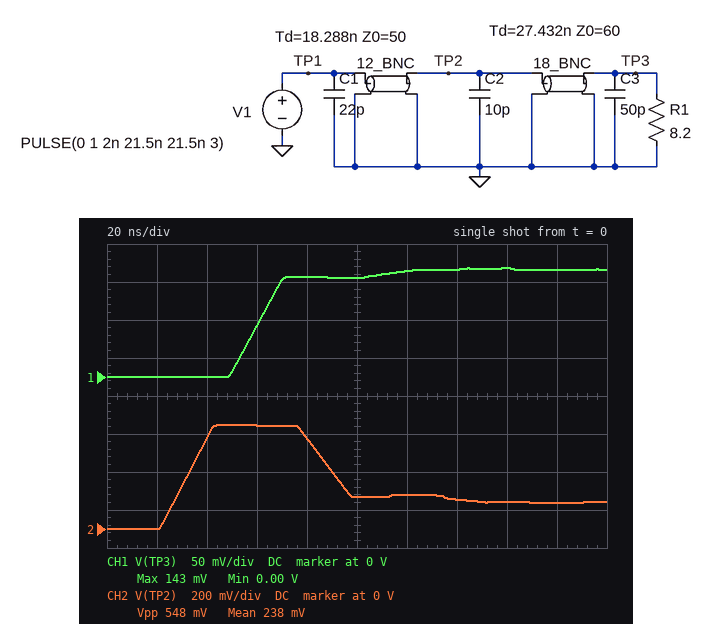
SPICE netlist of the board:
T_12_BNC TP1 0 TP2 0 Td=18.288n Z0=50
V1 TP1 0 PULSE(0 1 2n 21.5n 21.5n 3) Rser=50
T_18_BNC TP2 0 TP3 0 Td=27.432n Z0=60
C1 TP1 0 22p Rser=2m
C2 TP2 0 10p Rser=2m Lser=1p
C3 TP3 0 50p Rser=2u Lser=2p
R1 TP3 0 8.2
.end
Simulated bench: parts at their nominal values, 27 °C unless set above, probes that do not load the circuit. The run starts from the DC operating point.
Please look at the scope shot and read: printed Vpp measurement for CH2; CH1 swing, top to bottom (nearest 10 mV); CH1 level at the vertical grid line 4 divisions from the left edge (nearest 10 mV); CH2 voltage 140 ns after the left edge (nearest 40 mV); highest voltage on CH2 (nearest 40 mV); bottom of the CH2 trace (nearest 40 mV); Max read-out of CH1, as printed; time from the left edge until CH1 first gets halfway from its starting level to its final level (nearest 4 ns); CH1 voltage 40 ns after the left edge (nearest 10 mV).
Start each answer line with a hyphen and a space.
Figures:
- 548 mV
- 140 mV
- 130 mV
- 160 mV
- 560 mV
- 0 V
- 143 mV
- 60 ns
- 0 V
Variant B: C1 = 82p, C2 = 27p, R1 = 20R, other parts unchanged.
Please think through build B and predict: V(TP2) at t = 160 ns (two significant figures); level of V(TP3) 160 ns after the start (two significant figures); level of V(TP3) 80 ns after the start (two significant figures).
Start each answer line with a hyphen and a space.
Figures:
- 280 mV
- 300 mV
- 270 mV
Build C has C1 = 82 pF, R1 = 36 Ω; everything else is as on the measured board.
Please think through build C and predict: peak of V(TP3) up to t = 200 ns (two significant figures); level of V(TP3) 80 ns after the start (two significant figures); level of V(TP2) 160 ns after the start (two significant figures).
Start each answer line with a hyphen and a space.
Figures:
- 430 mV
- 410 mV
- 420 mV
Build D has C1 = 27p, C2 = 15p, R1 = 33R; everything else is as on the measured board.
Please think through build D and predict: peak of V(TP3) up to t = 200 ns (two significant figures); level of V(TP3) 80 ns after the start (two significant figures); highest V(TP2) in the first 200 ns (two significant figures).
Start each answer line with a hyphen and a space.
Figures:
- 400 mV
- 390 mV
- 550 mV
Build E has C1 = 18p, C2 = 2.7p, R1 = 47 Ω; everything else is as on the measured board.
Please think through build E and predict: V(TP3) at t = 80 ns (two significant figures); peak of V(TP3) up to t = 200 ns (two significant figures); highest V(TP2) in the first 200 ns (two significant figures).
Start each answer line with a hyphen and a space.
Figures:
- 480 mV
- 490 mV
- 550 mV
